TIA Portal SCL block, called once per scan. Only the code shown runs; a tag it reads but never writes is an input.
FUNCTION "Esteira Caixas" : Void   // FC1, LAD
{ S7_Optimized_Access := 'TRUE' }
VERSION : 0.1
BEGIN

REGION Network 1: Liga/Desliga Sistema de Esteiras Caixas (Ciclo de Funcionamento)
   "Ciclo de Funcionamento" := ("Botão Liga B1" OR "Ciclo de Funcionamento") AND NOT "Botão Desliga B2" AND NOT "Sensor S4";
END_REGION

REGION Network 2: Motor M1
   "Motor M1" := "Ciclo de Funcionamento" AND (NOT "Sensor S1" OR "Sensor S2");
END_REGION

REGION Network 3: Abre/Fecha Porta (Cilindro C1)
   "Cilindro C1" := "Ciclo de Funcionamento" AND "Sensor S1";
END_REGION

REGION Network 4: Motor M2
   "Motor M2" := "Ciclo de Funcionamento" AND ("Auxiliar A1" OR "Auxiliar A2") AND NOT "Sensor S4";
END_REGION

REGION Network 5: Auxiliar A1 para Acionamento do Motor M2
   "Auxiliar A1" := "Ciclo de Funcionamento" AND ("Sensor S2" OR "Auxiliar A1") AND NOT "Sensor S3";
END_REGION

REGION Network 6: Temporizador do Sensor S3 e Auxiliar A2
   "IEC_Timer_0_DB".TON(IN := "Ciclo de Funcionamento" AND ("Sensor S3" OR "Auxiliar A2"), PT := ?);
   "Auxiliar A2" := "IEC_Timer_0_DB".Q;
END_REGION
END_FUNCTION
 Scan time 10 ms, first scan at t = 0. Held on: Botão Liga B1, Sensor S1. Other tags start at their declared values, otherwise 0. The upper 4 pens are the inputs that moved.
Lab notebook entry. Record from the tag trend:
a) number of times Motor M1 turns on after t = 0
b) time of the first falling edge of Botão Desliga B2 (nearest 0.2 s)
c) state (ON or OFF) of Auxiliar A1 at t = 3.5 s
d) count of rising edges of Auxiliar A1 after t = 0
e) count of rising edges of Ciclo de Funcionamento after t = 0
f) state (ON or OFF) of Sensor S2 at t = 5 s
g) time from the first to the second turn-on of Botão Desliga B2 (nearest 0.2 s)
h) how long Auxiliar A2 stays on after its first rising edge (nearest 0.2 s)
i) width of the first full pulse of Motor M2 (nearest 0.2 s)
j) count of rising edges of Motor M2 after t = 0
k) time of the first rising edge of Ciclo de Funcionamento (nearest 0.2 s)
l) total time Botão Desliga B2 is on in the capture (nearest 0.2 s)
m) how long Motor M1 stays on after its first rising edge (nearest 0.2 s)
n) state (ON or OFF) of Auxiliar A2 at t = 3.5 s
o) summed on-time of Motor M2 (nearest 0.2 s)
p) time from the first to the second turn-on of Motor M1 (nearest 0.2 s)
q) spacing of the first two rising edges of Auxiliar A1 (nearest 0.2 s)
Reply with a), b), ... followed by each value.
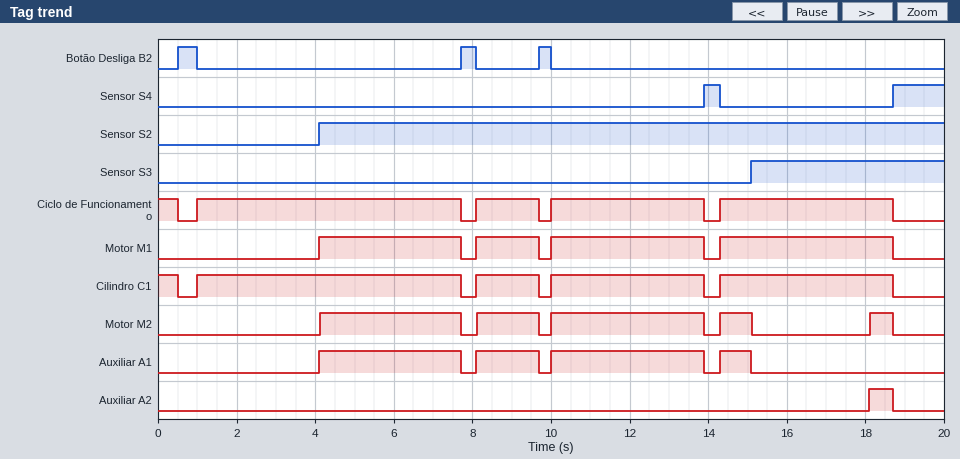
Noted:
a) 4
b) 1.0 s
c) OFF
d) 4
e) 4
f) ON
g) 7.2 s
h) 0.6 s
i) 3.6 s
j) 5
k) 1.0 s
l) 1.2 s
m) 3.6 s
n) OFF
o) 10.4 s
p) 4.0 s
q) 4.0 s
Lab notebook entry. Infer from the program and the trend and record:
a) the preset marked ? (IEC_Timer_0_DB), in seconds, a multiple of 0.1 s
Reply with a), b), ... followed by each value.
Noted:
a) 3.0 s
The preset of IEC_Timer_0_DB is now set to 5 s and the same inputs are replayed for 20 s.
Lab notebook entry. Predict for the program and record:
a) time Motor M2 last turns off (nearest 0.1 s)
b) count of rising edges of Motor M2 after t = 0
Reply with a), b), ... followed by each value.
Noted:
a) 15.1 s
b) 4
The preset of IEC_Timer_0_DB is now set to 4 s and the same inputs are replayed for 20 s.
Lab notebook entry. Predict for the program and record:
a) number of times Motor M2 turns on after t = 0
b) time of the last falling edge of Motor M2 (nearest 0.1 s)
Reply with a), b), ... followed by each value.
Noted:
a) 4
b) 15.1 s
